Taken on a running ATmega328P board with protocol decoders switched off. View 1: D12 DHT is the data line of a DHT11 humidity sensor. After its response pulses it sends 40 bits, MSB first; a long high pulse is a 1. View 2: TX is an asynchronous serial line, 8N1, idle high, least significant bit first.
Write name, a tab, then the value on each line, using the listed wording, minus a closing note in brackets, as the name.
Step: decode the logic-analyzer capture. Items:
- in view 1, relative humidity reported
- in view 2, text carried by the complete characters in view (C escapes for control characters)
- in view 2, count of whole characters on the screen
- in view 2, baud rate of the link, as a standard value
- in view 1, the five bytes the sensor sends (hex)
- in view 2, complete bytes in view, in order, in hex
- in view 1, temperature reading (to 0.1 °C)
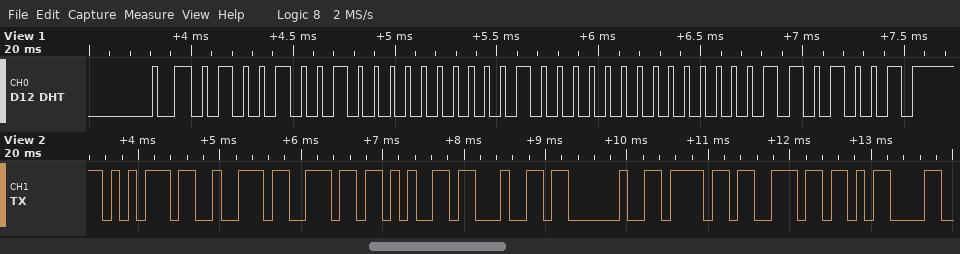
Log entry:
in view 1, relative humidity reported	73 %
in view 2, text carried by the complete characters in view	"urned on\r"
in view 2, count of whole characters on the screen	9
in view 2, baud rate of the link, as a standard value	9600 baud
in view 1, the five bytes the sensor sends	49 00 20 00 69
in view 2, complete bytes in view, in order, in hex	75 72 6E 65 64 20 6F 6E 0D
in view 1, temperature reading	32.0 °C
